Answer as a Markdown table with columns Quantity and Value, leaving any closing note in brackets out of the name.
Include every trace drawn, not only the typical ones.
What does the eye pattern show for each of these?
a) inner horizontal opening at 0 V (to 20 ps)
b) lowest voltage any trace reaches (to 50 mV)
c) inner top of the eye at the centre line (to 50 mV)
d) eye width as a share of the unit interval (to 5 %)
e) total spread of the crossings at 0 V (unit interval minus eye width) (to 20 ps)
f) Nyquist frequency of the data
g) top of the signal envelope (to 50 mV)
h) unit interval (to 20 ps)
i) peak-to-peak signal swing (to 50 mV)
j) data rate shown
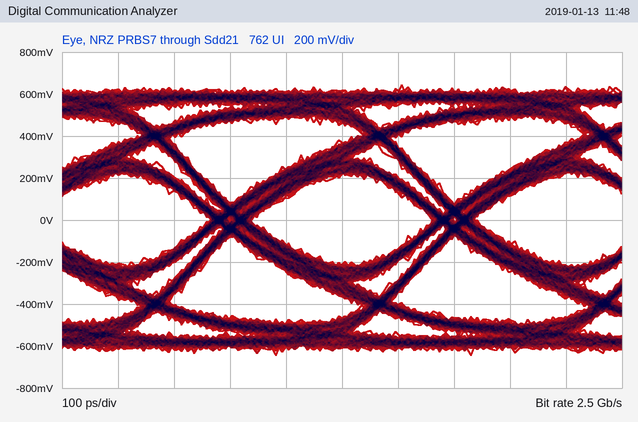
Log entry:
| Quantity | Value |
|---|---|
| inner horizontal opening at 0 V | 320 ps |
| lowest voltage any trace reaches | -650 mV |
| inner top of the eye at the centre line | 200 mV |
| eye width as a share of the unit interval | 80 % |
| total spread of the crossings at 0 V (unit interval minus eye width) | 80 ps |
| Nyquist frequency of the data | 1.25 GHz |
| top of the signal envelope | 650 mV |
| unit interval | 400 ps |
| peak-to-peak signal swing | 1.30 V |
| data rate shown | 2.5 Gb/s |
